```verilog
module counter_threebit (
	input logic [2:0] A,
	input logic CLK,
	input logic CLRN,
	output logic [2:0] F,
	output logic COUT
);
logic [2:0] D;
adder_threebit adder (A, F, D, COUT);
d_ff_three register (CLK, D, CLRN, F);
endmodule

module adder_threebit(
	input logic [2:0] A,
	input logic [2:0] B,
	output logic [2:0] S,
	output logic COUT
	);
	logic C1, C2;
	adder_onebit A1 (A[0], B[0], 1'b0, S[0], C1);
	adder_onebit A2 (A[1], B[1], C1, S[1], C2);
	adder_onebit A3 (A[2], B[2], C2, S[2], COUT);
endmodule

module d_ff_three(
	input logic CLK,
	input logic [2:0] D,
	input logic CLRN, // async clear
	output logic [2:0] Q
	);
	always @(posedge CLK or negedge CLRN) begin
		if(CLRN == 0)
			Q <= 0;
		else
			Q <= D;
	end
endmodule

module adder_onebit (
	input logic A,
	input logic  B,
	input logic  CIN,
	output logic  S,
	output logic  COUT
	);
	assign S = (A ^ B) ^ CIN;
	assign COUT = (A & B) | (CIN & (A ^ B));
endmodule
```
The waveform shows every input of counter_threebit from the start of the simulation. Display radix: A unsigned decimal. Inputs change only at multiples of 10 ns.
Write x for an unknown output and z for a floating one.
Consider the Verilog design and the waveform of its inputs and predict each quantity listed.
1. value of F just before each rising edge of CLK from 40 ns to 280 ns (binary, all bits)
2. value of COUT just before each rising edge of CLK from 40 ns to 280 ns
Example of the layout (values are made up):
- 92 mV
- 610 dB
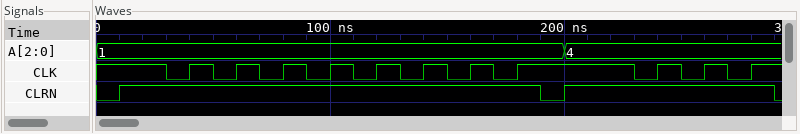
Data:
- 000, 001, 010, 011, 100, 101, 110, 111, 000, 100, 000
- 0 0 0 0 0 0 0 1 0 1 0
